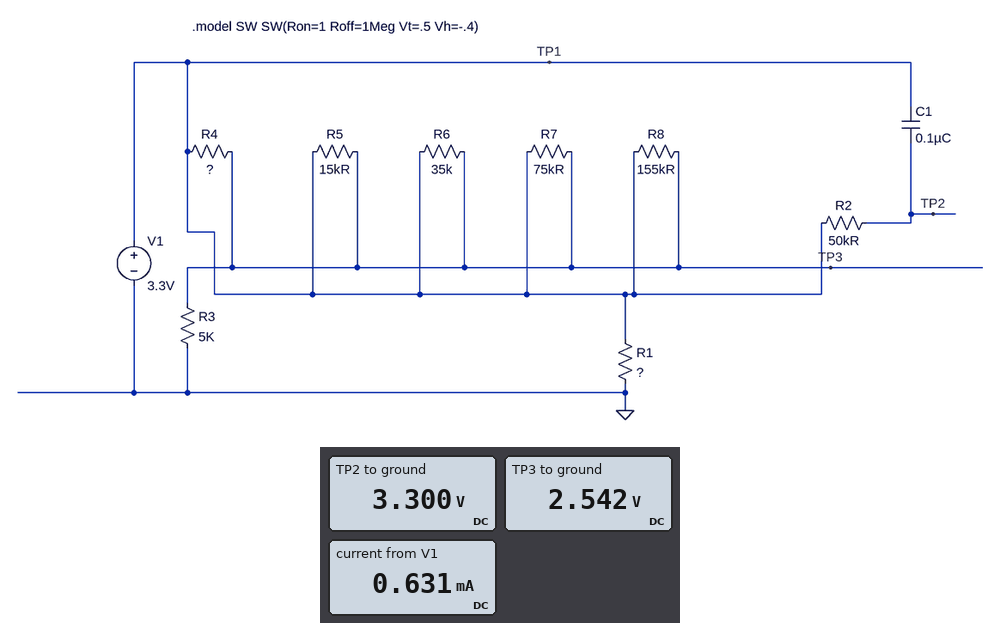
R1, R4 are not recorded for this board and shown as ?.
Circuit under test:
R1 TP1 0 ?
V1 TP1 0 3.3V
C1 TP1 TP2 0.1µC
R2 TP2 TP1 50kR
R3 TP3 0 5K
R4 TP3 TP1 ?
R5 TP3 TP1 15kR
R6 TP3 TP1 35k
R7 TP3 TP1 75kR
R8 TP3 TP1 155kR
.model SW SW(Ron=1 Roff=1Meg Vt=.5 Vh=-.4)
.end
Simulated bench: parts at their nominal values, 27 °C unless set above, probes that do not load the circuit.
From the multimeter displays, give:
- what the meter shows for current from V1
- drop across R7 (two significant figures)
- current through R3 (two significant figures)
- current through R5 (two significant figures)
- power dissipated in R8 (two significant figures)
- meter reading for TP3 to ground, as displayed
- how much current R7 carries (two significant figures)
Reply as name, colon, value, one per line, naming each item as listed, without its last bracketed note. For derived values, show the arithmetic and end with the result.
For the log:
what the meter shows for current from V1: 0.631 mA
drop across R7: 3.3 V - 2.542 V = 760 mV
current through R3: (2.542 V) / 5 kΩ = 510 µA
current through R5: (3.3 V - 2.542 V) / 15 kΩ = 51 µA
power dissipated in R8: (3.3 V - 2.542 V)^2 / 155 kΩ = 3.7 µW
meter reading for TP3 to ground, as displayed: 2.542 V
how much current R7 carries: (3.3 V - 2.542 V) / 75 kΩ = 10 µA
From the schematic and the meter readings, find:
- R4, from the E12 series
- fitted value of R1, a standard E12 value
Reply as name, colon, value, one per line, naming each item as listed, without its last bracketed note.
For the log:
R4, from the E12 series: 1.8 kΩ
fitted value of R1, a standard E12 value: 27 kΩ
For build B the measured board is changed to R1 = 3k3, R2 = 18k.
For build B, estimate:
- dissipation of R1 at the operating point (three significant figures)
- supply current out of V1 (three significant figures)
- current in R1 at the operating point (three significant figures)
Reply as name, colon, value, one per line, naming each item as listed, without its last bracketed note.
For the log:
dissipation of R1 at the operating point: 3.30 mW
supply current out of V1: 1.51 mA
current in R1 at the operating point: 1.00 mA
